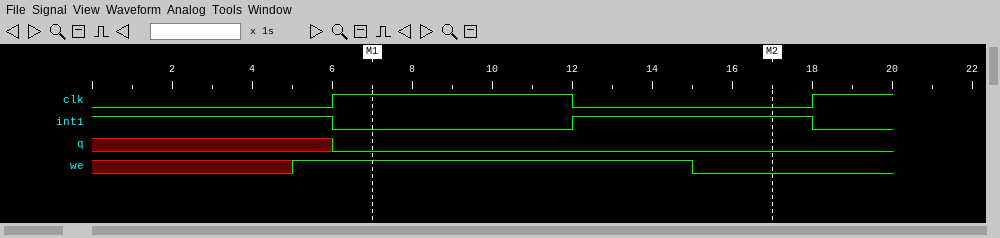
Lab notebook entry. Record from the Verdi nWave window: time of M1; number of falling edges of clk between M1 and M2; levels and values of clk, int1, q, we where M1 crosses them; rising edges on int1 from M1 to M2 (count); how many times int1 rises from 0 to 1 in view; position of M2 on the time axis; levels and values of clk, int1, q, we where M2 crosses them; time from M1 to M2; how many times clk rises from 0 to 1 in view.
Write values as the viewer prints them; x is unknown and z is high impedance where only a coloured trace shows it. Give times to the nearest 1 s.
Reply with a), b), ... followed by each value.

a) 7 s
b) 1
c) clk=1, int1=0, q=0, we=1
d) 1
e) 1
f) 17 s
g) clk=0, int1=1, q=0, we=0
h) 10 s
i) 2
